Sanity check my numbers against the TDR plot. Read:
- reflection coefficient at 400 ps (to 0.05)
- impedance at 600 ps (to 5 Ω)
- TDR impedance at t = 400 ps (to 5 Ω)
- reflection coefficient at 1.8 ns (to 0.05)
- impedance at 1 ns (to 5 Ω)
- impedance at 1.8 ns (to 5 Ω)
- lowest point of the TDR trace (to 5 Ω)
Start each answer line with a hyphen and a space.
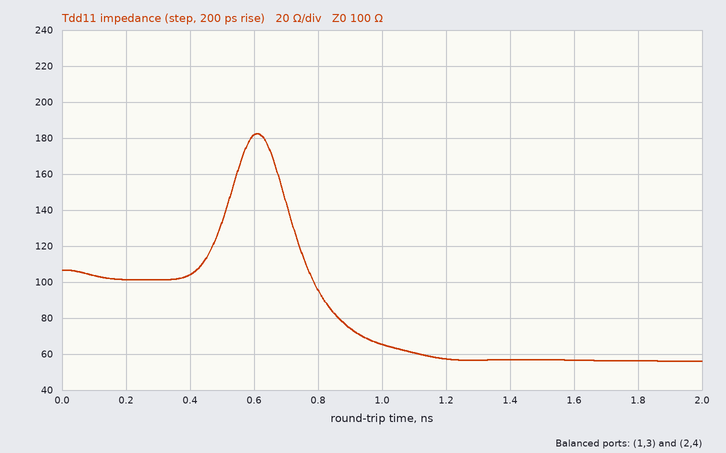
- 0.00
- 180 Ω
- 105 Ω
- -0.30
- 65 Ω
- 55 Ω
- 55 Ω
